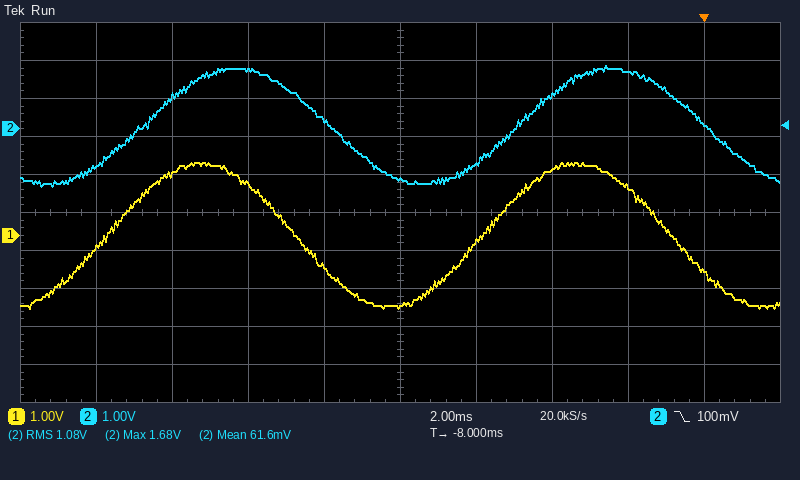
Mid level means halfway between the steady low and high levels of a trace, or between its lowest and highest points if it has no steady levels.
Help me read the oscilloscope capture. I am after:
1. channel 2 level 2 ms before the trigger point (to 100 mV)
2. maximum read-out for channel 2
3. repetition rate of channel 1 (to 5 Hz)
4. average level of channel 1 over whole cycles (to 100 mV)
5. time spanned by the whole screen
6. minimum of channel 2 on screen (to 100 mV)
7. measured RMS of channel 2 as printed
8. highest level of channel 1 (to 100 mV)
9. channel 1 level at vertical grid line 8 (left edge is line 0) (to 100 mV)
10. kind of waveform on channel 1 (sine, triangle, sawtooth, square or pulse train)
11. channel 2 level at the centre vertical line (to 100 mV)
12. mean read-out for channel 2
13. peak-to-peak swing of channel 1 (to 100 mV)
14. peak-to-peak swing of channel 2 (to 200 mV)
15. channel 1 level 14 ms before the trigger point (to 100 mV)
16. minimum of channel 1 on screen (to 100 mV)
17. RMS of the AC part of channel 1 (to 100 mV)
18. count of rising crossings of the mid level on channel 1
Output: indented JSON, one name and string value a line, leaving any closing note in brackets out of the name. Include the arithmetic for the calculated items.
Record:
{
  "channel 2 level 2 ms before the trigger point": "1.5 V",
  "maximum read-out for channel 2": "1.68 V",
  "repetition rate of channel 1": "100 Hz",
  "average level of channel 1 over whole cycles": "(1.9 V + (-1.9 V)) / 2 ≈ 0.0 V",
  "time spanned by the whole screen": "20 ms",
  "minimum of channel 2 on screen": "-1.5 V",
  "measured RMS of channel 2 as printed": "1.08 V",
  "highest level of channel 1": "1.9 V",
  "channel 1 level at vertical grid line 8 (left edge is line 0)": "1.3 V",
  "kind of waveform on channel 1": "sine",
  "channel 2 level at the centre vertical line": "-1.3 V",
  "mean read-out for channel 2": "61.6 mV",
  "peak-to-peak swing of channel 1": "1.9 V − (-1.9 V) = 3.8 V",
  "peak-to-peak swing of channel 2": "3.2 V",
  "channel 1 level 14 ms before the trigger point": "1.6 V",
  "minimum of channel 1 on screen": "-1.9 V",
  "RMS of the AC part of channel 1": "3.8 V / (2√2) ≈ 1.3 V",
  "count of rising crossings of the mid level on channel 1": "2"
}
